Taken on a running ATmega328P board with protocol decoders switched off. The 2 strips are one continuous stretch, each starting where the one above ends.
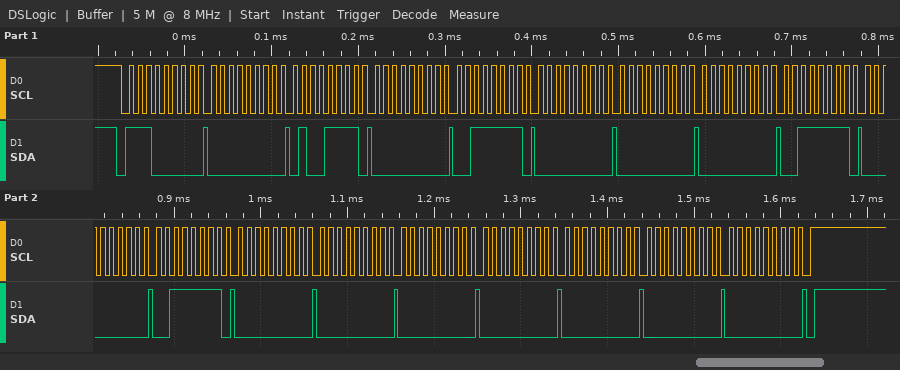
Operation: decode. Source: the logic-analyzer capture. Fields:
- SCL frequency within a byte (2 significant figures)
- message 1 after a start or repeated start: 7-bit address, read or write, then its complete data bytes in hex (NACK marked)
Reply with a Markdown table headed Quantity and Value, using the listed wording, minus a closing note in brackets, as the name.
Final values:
| Quantity | Value |
|---|---|
| SCL frequency within a byte | 100 kHz |
| message 1 after a start or repeated start: 7-bit address, read or write, then its complete data bytes in hex | 0x70 write: 00 4F 00 3F 00 00 00 3F 00 3F 00 00 00 00 00 00 00 |
